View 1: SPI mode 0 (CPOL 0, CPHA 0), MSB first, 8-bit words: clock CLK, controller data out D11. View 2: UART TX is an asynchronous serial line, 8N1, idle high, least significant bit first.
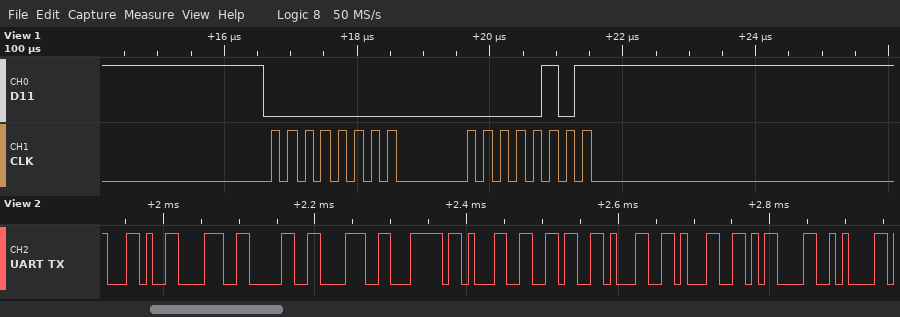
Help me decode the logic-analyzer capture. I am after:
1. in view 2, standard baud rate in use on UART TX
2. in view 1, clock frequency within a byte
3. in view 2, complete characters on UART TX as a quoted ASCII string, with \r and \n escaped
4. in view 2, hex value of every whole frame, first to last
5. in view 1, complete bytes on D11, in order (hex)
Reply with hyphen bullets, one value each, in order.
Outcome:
- 115200 baud
- 4 MHz
- ",808|1611\r\n"
- 2C 38 30 38 7C 31 36 31 31 0D 0A
- 00 05
